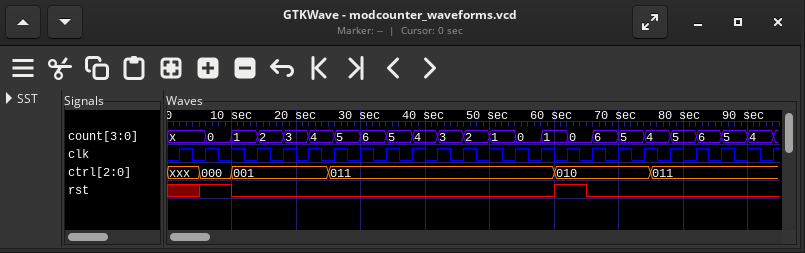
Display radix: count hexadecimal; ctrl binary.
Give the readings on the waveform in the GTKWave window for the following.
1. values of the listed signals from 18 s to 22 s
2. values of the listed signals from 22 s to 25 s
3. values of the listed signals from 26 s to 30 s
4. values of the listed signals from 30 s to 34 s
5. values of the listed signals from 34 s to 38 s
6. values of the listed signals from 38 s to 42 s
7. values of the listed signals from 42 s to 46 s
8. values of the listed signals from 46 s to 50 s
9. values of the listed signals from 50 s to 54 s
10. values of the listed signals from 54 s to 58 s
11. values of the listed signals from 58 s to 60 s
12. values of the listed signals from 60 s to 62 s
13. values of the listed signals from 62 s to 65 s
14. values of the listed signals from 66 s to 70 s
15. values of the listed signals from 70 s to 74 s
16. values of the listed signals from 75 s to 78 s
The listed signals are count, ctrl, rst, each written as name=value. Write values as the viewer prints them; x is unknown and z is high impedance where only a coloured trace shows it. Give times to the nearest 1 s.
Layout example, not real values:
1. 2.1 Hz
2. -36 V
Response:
1. count=3, ctrl=001, rst=0
2. count=4, ctrl=001, rst=0
3. count=5, ctrl=011, rst=0
4. count=6, ctrl=011, rst=0
5. count=5, ctrl=011, rst=0
6. count=4, ctrl=011, rst=0
7. count=3, ctrl=011, rst=0
8. count=2, ctrl=011, rst=0
9. count=1, ctrl=011, rst=0
10. count=0, ctrl=011, rst=0
11. count=1, ctrl=011, rst=0
12. count=1, ctrl=010, rst=1
13. count=0, ctrl=010, rst=1
14. count=6, ctrl=010, rst=0
15. count=5, ctrl=010, rst=0
16. count=4, ctrl=011, rst=0
